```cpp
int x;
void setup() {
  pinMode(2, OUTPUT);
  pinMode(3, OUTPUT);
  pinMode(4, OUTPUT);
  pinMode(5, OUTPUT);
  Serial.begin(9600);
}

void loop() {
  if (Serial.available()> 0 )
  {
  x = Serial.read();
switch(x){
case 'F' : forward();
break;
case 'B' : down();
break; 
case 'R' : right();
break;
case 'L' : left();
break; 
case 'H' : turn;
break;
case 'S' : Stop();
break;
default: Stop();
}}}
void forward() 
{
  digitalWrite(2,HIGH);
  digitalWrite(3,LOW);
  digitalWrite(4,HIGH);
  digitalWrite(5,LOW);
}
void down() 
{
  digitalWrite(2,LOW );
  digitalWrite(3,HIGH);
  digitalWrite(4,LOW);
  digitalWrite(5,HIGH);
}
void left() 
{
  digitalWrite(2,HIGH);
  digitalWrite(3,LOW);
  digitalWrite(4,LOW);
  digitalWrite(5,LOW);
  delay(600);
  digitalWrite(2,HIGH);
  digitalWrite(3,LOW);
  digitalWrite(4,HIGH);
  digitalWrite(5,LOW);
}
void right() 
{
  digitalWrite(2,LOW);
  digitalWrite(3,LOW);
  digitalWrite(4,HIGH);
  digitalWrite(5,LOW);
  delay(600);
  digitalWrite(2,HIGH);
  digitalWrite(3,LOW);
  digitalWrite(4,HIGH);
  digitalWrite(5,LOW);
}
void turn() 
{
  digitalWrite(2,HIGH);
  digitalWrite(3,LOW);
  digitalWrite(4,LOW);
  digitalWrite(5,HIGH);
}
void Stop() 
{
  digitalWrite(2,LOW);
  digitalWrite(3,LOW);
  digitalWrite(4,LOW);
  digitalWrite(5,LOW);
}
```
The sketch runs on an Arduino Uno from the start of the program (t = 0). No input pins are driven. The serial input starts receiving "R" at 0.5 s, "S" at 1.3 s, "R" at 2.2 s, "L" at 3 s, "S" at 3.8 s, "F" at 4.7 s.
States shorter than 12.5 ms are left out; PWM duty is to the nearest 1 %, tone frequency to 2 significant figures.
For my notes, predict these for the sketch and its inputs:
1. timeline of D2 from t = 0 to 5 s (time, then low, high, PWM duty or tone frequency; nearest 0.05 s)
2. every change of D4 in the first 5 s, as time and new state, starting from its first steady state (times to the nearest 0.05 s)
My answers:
0 s low; 1.1 s high; 1.3 s low; 2.8 s high; 3.8 s low; 4.7 s high
0 s low; 0.5 s high; 1.3 s low; 2.2 s high; 3 s low; 3.6 s high; 3.8 s low; 4.7 s high
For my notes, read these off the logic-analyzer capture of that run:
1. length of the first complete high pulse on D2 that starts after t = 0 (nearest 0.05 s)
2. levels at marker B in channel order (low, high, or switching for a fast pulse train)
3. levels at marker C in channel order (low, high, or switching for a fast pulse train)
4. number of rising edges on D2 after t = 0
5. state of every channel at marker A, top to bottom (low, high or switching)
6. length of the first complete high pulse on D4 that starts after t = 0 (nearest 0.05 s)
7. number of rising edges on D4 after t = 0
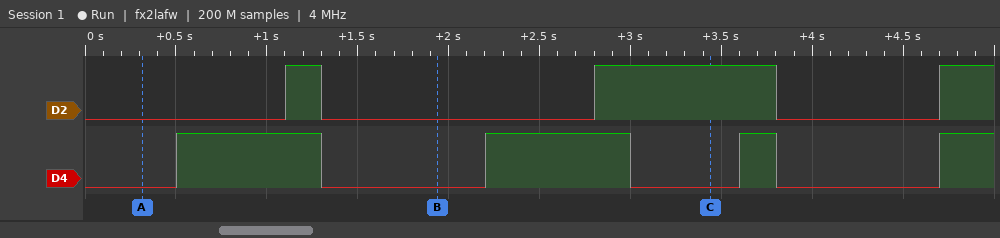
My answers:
0.20 s
D2 low, D4 low
D2 high, D4 low
3
D2 low, D4 low
0.80 s
4
